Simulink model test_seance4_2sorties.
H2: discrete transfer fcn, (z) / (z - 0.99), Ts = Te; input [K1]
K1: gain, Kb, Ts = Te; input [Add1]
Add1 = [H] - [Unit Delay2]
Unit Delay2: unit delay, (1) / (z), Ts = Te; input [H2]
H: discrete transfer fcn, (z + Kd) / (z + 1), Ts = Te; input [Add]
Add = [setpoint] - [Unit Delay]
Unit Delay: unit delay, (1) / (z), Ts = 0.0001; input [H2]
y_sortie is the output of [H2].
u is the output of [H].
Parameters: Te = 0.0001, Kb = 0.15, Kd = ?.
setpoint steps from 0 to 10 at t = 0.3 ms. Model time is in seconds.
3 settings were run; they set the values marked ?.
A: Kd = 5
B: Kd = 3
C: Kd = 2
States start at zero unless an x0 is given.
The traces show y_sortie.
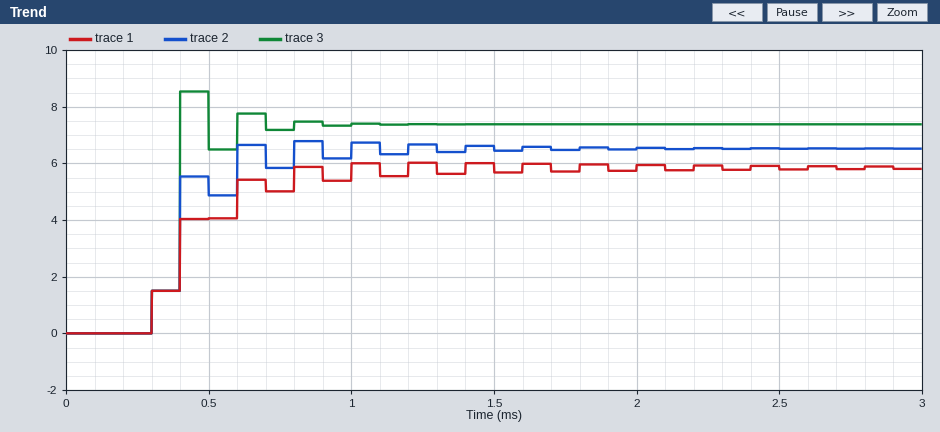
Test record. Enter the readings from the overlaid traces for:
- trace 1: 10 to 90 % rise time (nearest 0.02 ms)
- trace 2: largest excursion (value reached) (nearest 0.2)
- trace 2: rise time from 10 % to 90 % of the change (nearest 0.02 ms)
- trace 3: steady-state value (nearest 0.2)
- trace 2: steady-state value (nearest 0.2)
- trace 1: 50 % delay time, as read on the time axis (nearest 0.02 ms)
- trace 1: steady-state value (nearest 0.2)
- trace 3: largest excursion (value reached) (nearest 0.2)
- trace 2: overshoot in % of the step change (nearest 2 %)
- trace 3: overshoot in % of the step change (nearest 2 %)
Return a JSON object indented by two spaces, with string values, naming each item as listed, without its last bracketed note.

{
  "trace 1: 10 to 90 % rise time": "0.30 ms",
  "trace 2: largest excursion (value reached)": "6.8",
  "trace 2: rise time from 10 % to 90 % of the change": "0.30 ms",
  "trace 3: steady-state value": "7.4",
  "trace 2: steady-state value": "6.6",
  "trace 1: 50 % delay time, as read on the time axis": "0.40 ms",
  "trace 1: steady-state value": "5.8",
  "trace 3: largest excursion (value reached)": "8.6",
  "trace 2: overshoot in % of the step change": "4 %",
  "trace 3: overshoot in % of the step change": "16 %"
}
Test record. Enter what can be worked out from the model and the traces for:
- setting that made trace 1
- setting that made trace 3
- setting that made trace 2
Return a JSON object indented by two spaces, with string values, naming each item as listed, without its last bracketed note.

{
  "setting that made trace 1": "C",
  "setting that made trace 3": "A",
  "setting that made trace 2": "B"
}
